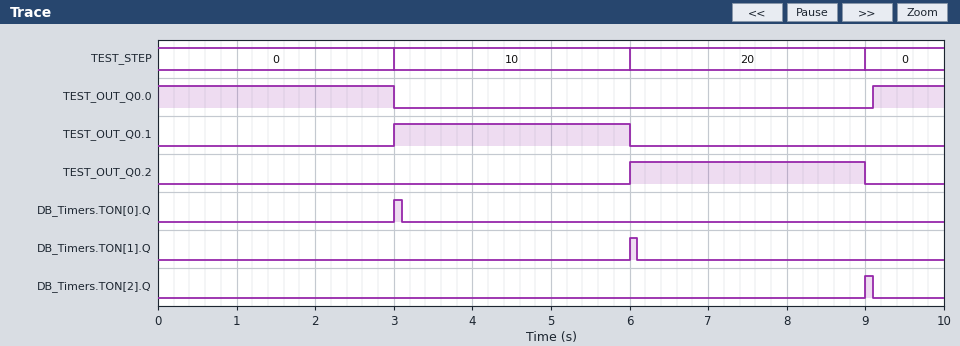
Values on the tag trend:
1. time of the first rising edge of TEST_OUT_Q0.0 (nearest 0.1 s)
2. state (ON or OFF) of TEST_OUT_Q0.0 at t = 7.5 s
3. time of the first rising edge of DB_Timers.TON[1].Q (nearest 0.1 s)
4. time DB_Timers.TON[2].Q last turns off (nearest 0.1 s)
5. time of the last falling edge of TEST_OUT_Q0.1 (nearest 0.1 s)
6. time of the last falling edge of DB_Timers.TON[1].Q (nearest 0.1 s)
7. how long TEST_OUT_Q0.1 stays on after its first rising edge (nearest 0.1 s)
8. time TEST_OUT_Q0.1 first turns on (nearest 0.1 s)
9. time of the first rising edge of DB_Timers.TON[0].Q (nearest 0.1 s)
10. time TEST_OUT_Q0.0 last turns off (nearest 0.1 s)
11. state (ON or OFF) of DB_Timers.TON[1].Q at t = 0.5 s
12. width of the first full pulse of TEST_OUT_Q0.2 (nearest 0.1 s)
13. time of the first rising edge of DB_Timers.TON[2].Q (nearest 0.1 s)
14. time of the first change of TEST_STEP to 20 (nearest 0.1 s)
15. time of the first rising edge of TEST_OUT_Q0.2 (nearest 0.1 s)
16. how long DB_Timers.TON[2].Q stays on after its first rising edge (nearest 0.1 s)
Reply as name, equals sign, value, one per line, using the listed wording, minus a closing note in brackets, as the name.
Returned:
time of the first rising edge of TEST_OUT_Q0.0 = 9.1 s
state (ON or OFF) of TEST_OUT_Q0.0 at t = 7.5 s = OFF
time of the first rising edge of DB_Timers.TON[1].Q = 6.0 s
time DB_Timers.TON[2].Q last turns off = 9.1 s
time of the last falling edge of TEST_OUT_Q0.1 = 6.0 s
time of the last falling edge of DB_Timers.TON[1].Q = 6.1 s
how long TEST_OUT_Q0.1 stays on after its first rising edge = 3.0 s
time TEST_OUT_Q0.1 first turns on = 3.0 s
time of the first rising edge of DB_Timers.TON[0].Q = 3.0 s
time TEST_OUT_Q0.0 last turns off = 3.0 s
state (ON or OFF) of DB_Timers.TON[1].Q at t = 0.5 s = OFF
width of the first full pulse of TEST_OUT_Q0.2 = 3.0 s
time of the first rising edge of DB_Timers.TON[2].Q = 9.0 s
time of the first change of TEST_STEP to 20 = 6.0 s
time of the first rising edge of TEST_OUT_Q0.2 = 6.0 s
how long DB_Timers.TON[2].Q stays on after its first rising edge = 0.1 s
